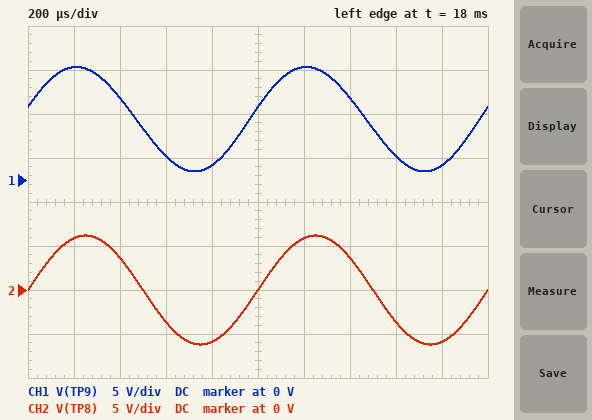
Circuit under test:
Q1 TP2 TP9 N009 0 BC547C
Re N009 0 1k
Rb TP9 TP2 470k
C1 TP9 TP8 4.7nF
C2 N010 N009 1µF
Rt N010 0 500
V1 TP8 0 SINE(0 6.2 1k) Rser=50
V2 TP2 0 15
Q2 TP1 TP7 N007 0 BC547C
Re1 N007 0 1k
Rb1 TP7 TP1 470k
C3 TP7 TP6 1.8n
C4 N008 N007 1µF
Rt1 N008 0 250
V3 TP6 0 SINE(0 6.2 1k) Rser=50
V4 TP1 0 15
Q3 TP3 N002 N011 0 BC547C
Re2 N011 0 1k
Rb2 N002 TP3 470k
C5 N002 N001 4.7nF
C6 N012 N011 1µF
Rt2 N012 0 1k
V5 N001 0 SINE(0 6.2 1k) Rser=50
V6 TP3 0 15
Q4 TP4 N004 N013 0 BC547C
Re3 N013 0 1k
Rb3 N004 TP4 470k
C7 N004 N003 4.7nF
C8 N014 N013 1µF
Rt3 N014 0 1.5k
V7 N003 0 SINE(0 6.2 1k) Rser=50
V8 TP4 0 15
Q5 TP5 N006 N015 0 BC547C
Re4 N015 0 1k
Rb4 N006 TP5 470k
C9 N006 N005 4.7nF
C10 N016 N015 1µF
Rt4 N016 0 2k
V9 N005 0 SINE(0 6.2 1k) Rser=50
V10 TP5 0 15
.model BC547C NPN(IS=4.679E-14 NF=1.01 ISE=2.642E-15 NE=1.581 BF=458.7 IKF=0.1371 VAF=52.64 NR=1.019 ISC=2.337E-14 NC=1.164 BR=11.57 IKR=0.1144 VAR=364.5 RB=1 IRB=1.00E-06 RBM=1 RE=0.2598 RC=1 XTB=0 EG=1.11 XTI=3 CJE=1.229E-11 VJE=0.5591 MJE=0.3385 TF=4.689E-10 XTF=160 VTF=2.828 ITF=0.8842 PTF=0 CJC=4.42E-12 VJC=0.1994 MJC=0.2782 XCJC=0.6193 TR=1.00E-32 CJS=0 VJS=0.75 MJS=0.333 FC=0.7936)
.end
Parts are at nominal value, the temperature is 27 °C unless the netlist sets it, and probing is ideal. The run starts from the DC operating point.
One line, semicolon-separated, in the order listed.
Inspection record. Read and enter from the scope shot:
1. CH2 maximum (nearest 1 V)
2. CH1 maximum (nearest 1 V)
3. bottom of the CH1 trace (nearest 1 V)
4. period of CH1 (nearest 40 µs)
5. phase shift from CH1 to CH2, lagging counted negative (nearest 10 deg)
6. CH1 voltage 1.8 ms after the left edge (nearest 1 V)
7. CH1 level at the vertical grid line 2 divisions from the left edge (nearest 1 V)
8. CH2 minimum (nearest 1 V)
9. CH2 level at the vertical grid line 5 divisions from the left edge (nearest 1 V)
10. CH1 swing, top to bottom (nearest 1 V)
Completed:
6 V; 13 V; 1 V; 1.00 ms; -10 deg; 2 V; 9 V; -6 V; 0 V; 12 V
